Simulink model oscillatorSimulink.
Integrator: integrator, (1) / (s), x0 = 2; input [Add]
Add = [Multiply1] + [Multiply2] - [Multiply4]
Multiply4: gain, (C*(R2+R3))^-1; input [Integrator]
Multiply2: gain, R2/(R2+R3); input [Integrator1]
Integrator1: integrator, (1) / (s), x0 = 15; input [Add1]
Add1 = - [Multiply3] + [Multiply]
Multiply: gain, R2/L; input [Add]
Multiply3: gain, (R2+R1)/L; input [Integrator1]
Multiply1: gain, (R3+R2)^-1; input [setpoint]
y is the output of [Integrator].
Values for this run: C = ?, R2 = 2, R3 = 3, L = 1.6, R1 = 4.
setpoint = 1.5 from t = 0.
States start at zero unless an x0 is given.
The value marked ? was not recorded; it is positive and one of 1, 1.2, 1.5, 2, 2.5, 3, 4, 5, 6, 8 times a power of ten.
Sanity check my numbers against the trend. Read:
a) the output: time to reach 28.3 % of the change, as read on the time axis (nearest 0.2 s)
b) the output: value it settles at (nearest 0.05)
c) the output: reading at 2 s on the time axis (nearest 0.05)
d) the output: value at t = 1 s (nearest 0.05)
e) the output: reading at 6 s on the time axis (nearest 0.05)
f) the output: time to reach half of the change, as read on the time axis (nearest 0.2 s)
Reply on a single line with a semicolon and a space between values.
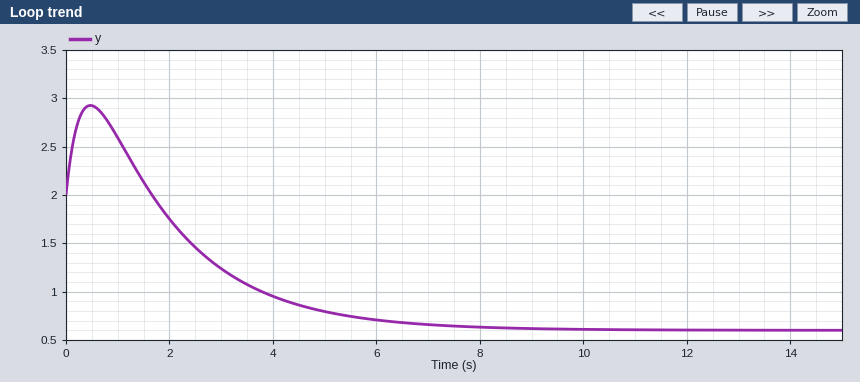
2.2 s; 0.60; 1.75; 2.60; 0.70; 2.8 s
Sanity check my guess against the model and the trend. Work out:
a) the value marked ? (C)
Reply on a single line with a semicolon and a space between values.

0.4
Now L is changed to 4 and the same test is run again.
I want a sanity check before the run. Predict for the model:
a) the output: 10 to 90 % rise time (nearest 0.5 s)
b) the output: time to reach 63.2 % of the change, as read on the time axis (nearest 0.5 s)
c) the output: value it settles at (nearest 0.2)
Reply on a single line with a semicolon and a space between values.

3.5 s; 5.0 s; 0.6
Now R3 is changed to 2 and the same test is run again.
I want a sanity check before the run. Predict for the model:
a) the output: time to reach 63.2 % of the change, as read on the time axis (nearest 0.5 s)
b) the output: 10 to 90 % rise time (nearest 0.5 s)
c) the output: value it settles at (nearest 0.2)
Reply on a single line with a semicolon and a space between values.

3.0 s; 3.0 s; 0.6
